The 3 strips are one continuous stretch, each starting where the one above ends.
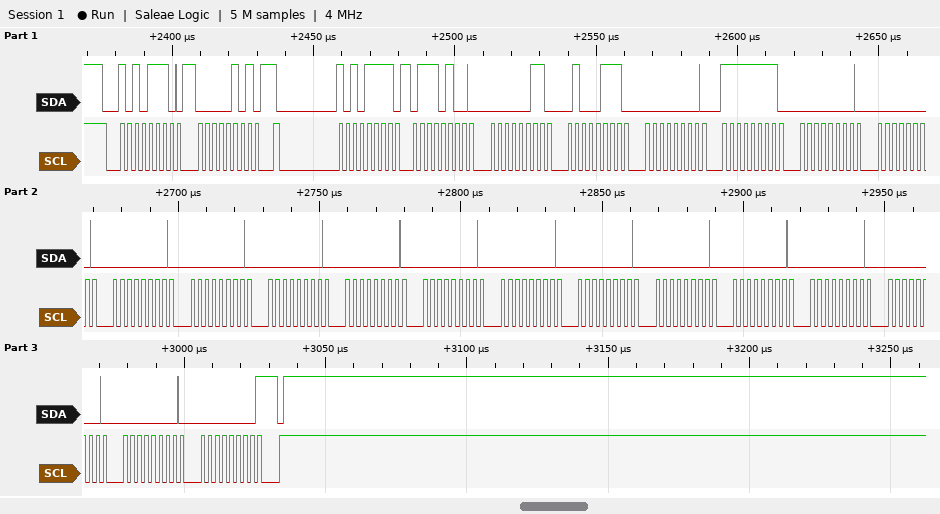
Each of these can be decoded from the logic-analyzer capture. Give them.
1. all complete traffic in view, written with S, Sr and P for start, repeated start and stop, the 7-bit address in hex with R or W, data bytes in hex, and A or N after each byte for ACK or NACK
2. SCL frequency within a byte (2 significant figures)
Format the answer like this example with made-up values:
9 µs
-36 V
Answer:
S 57W A 05 A Sr 57R A 74 A 03 A 47 A 00 A FF A 00 A 00 A 00 A 00 A 00 A 00 A 00 A 00 A 00 A 00 A 00 A 00 A 00 A 00 A 00 N P
400 kHz
